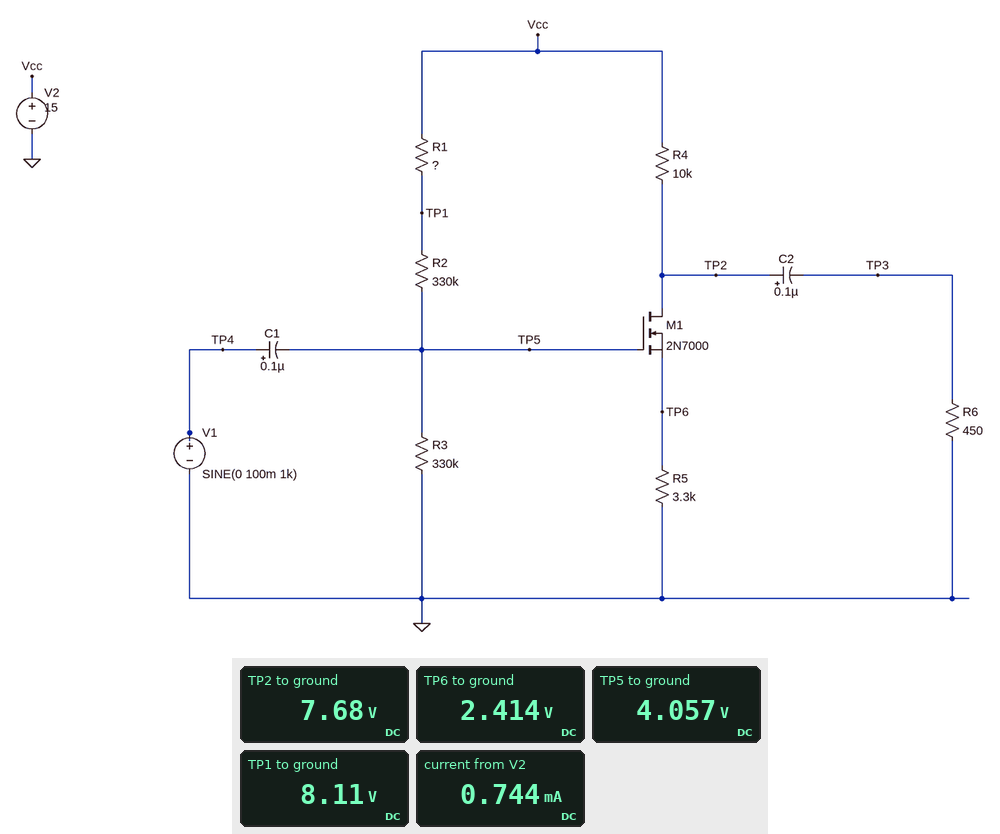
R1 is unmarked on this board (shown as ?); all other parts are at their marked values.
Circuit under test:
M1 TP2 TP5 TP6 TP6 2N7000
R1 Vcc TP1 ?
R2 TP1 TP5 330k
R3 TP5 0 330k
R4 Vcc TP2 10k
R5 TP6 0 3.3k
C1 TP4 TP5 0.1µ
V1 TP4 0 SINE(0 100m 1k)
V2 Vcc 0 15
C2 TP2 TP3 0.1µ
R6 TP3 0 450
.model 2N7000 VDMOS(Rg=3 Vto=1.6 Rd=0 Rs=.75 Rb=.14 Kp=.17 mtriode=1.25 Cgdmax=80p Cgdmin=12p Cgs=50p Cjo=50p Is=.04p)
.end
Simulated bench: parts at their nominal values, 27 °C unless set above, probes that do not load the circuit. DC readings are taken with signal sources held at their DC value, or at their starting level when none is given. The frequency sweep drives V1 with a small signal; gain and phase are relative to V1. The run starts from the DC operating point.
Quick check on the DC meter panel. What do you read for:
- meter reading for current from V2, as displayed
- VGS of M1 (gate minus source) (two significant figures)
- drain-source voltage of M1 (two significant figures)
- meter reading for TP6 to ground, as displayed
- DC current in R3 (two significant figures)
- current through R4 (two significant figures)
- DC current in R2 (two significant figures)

0.744 mA
1.6 V
5.3 V
2.414 V
12 µA
730 µA
12 µA
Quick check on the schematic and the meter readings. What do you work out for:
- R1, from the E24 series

560 kΩ
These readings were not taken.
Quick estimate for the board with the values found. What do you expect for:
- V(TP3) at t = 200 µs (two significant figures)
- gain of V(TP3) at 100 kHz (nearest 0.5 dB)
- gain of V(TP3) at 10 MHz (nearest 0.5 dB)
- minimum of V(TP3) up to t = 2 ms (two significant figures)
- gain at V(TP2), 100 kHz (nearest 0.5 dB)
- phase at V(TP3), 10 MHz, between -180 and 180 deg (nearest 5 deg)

-11 mV
-18.0 dB
-4.0 dB
-12 mV
-18.0 dB
75 deg
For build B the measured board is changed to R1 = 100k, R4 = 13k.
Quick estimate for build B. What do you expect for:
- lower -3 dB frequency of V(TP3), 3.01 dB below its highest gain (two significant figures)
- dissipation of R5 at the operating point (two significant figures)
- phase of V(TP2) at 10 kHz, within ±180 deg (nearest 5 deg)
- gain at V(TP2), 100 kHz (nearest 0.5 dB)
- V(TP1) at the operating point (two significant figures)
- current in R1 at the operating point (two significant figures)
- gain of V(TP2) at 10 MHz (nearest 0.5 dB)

3.2 MHz
2.8 mW
75 deg
-30.0 dB
13 V
20 µA
-0.5 dB
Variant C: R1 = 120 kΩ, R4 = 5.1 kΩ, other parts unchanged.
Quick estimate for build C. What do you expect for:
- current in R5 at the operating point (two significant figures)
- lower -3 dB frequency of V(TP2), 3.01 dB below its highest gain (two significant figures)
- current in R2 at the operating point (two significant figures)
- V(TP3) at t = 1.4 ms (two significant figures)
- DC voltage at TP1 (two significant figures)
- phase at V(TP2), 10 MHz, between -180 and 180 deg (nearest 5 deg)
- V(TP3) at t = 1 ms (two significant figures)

1.4 mA
7.9 Hz
19 µA
-3.7 mV
13 V
65 deg
-2.8 mV
